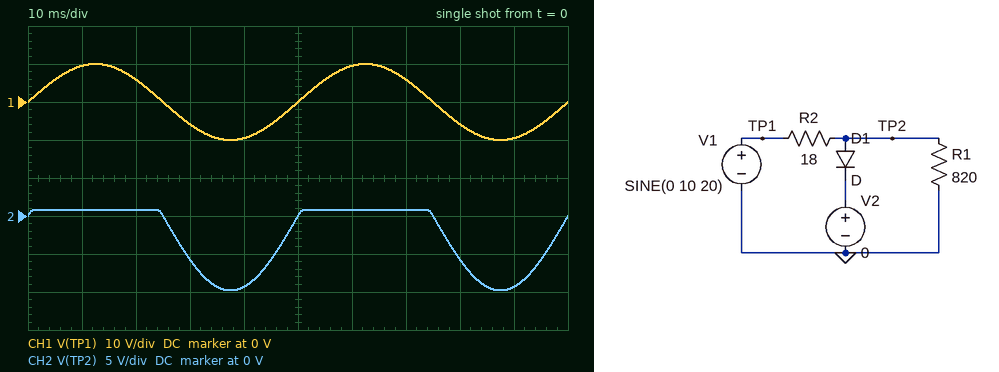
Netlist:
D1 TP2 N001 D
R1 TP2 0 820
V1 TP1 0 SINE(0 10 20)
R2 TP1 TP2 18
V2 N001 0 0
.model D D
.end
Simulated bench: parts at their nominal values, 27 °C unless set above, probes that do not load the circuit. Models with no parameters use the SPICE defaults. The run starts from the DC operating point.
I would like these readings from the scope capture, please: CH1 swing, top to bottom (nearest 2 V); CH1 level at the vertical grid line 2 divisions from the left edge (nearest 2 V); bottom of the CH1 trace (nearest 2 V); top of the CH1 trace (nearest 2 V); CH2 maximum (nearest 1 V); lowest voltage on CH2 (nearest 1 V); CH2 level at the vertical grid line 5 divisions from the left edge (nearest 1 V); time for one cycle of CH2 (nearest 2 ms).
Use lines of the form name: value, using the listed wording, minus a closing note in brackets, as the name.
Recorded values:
CH1 swing, top to bottom: 20 V
CH1 level at the vertical grid line 2 divisions from the left edge: 6 V
bottom of the CH1 trace: -10 V
top of the CH1 trace: 10 V
CH2 maximum: 1 V
lowest voltage on CH2: -10 V
CH2 level at the vertical grid line 5 divisions from the left edge: 0 V
time for one cycle of CH2: 50 ms
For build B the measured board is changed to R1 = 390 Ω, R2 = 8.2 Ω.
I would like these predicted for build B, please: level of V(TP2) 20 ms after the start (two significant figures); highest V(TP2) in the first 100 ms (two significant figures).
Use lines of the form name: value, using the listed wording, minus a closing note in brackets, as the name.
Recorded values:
level of V(TP2) 20 ms after the start: 820 mV
highest V(TP2) in the first 100 ms: 840 mV
